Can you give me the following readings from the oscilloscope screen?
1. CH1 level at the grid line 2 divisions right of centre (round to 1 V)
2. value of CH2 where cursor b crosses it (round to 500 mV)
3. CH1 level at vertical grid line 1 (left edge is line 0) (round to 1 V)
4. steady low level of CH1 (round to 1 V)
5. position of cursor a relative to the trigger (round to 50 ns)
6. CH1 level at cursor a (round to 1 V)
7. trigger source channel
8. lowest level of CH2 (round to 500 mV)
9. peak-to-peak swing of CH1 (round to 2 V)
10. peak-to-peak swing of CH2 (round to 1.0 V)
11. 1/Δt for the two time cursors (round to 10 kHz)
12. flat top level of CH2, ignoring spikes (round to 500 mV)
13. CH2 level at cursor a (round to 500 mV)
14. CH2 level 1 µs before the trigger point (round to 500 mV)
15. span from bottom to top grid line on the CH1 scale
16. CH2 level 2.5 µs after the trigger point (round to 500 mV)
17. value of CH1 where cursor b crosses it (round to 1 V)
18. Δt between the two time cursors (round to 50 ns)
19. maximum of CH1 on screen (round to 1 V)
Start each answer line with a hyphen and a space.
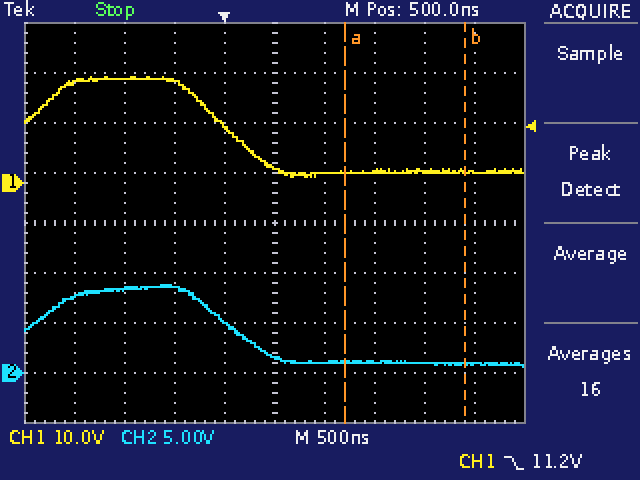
- 2 V
- 1.0 V
- 20 V
- 2 V
- +1.20 µs
- 2 V
- CH1
- 500 mV
- 20 V
- 8.0 V
- 830 kHz
- 8.5 V
- 1.0 V
- 8.5 V
- 80 V
- 1.0 V
- 2 V
- 1.20 µs
- 21 V
